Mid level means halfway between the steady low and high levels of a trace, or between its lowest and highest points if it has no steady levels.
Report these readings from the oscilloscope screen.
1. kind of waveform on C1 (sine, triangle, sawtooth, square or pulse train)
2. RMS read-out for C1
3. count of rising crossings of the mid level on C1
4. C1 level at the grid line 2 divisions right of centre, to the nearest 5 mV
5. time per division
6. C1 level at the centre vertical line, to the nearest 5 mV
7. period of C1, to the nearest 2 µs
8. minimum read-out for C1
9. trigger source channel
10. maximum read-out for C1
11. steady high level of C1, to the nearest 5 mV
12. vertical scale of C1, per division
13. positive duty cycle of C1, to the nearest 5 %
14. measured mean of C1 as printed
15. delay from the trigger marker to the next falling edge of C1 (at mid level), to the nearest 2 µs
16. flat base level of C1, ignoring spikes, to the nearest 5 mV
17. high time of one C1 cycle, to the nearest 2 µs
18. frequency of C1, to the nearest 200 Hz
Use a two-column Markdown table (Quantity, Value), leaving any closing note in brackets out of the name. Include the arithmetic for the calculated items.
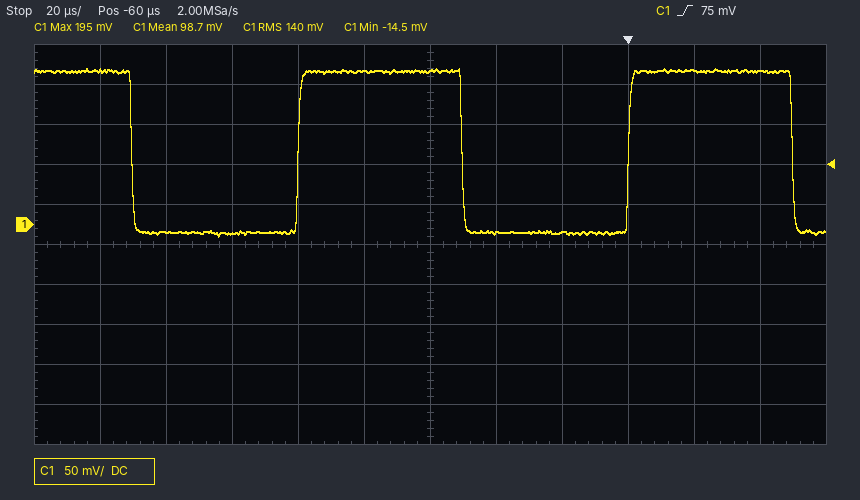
| Quantity | Value |
|---|---|
| kind of waveform on C1 | square |
| RMS read-out for C1 | 140 mV |
| count of rising crossings of the mid level on C1 | 2 |
| C1 level at the grid line 2 divisions right of centre, to the nearest 5 mV | -10 mV |
| time per division | 20 µs |
| C1 level at the centre vertical line, to the nearest 5 mV | 190 mV |
| period of C1, to the nearest 2 µs | 100 µs |
| minimum read-out for C1 | -14.5 mV |
| trigger source channel | C1 |
| maximum read-out for C1 | 195 mV |
| steady high level of C1, to the nearest 5 mV | 190 mV |
| vertical scale of C1, per division | 50 mV |
| positive duty cycle of C1, to the nearest 5 % | 50 µs / 100 µs ≈ 50 % |
| measured mean of C1 as printed | 98.7 mV |
| delay from the trigger marker to the next falling edge of C1 (at mid level), to the nearest 2 µs | 50 µs |
| flat base level of C1, ignoring spikes, to the nearest 5 mV | -10 mV |
| high time of one C1 cycle, to the nearest 2 µs | 50 µs |
| frequency of C1, to the nearest 200 Hz | 1 / 100 µs ≈ 10.0 kHz |
